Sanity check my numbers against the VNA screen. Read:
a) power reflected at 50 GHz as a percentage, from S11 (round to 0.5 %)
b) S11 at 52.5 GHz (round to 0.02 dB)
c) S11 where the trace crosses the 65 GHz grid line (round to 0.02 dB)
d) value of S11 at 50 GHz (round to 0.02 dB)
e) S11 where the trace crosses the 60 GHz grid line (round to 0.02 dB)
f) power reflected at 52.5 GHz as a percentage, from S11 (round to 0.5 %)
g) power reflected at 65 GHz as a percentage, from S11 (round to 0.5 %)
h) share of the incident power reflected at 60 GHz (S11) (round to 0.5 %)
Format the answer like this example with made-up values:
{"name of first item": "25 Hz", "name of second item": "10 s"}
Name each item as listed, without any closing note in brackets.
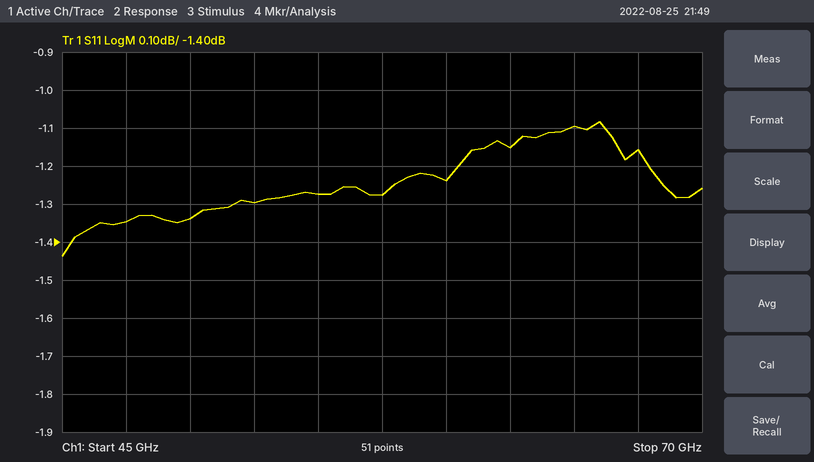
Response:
{"power reflected at 50 GHz as a percentage, from S11": "73.5 %", "S11 at 52.5 GHz": "-1.30 dB", "S11 where the trace crosses the 65 GHz grid line": "-1.10 dB", "value of S11 at 50 GHz": "-1.34 dB", "S11 where the trace crosses the 60 GHz grid line": "-1.24 dB", "power reflected at 52.5 GHz as a percentage, from S11": "74.0 %", "power reflected at 65 GHz as a percentage, from S11": "77.5 %", "share of the incident power reflected at 60 GHz (S11)": "75.0 %"}
